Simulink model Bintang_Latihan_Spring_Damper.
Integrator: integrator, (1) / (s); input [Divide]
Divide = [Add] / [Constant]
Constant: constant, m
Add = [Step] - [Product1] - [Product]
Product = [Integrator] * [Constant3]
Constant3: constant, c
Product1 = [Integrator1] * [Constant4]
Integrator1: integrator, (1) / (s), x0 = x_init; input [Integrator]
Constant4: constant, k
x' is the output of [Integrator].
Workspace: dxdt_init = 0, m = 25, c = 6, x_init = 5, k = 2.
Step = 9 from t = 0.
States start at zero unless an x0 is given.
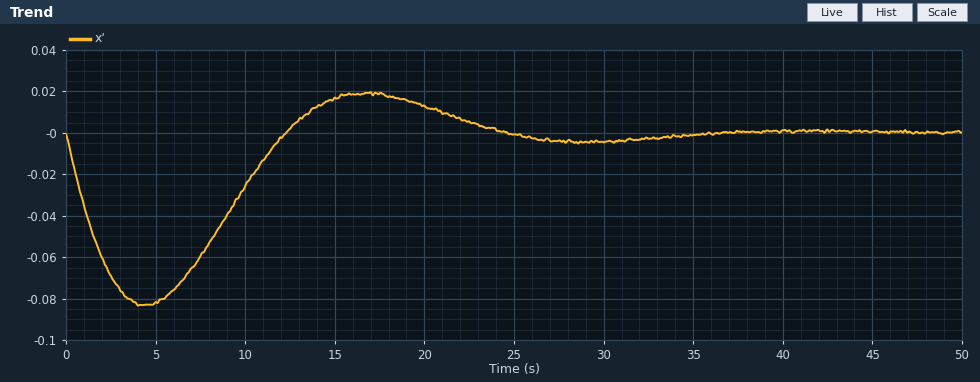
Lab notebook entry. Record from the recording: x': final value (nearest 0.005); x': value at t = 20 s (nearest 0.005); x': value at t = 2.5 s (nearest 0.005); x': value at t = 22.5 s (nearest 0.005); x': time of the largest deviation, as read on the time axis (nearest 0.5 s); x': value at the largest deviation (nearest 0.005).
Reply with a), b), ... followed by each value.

a) 0.000
b) 0.015
c) -0.070
d) 0.005
e) 4.5 s
f) -0.085
